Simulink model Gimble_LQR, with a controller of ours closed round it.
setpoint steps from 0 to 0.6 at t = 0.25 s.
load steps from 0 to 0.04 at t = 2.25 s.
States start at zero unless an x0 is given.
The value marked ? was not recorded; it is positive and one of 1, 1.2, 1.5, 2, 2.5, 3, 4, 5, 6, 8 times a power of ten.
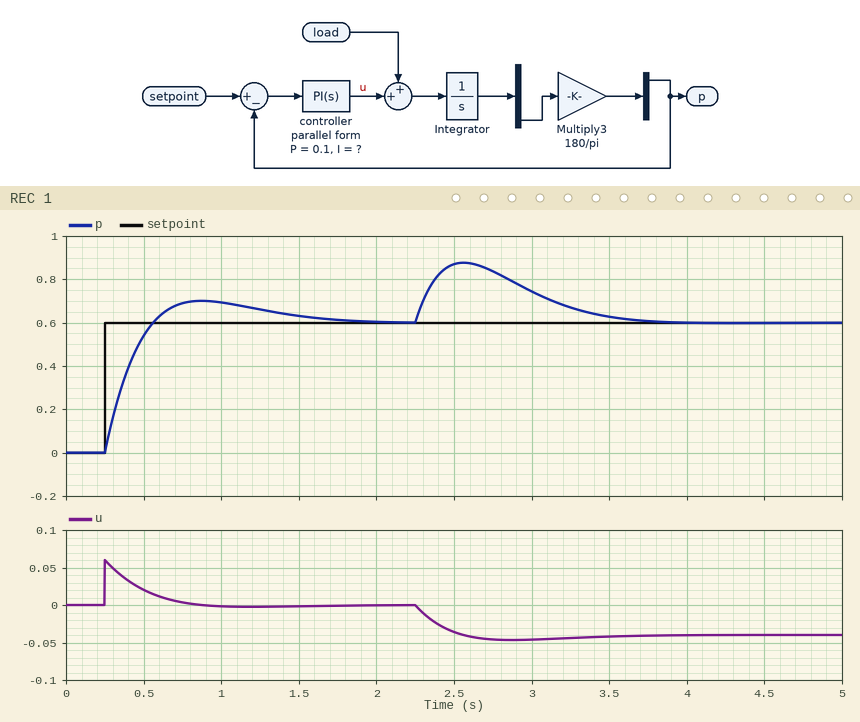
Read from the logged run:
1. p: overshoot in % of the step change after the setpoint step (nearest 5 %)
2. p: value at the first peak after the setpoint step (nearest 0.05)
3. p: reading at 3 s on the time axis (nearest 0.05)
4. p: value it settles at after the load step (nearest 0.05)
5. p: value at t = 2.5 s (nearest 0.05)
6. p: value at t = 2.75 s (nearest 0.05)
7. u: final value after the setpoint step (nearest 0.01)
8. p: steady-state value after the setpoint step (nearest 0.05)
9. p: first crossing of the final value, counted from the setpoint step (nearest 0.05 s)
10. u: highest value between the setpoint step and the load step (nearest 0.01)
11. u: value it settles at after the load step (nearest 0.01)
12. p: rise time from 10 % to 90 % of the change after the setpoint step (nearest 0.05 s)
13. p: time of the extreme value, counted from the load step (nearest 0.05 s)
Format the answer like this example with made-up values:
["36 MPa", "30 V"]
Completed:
["15 %", "0.70", "0.75", "0.60", "0.85", "0.85", "0.00", "0.60", "0.30 s", "0.06", "-0.04", "0.25 s", "0.30 s"]
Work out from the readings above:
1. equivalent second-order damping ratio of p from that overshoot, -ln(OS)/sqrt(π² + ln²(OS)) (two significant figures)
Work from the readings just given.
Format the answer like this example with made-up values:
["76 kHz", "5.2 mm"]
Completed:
["0.52"]
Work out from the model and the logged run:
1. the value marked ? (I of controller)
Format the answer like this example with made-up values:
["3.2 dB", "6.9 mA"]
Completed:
["0.2"]
